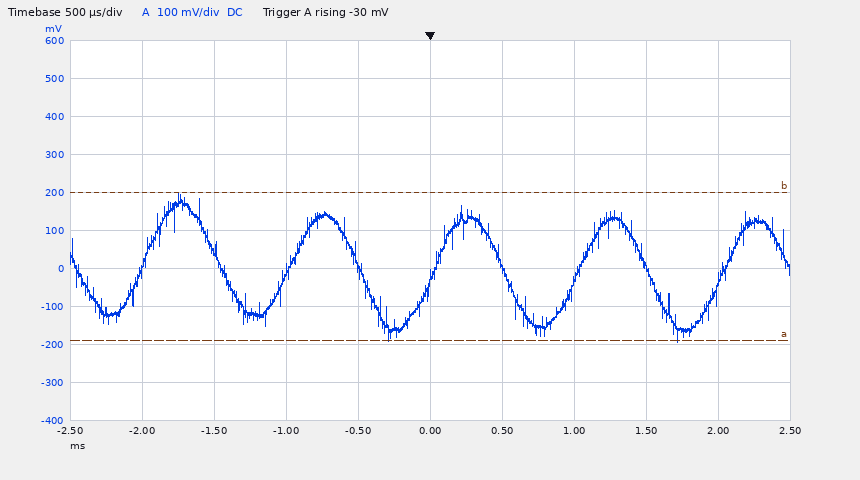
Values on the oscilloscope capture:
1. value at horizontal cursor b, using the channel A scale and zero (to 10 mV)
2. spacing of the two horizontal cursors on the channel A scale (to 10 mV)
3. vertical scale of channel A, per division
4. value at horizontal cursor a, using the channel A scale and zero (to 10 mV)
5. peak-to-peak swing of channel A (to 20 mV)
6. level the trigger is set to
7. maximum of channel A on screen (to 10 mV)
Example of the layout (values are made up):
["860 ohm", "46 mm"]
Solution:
["200 mV", "390 mV", "100 mV", "-190 mV", "400 mV", "-30 mV", "200 mV"]
